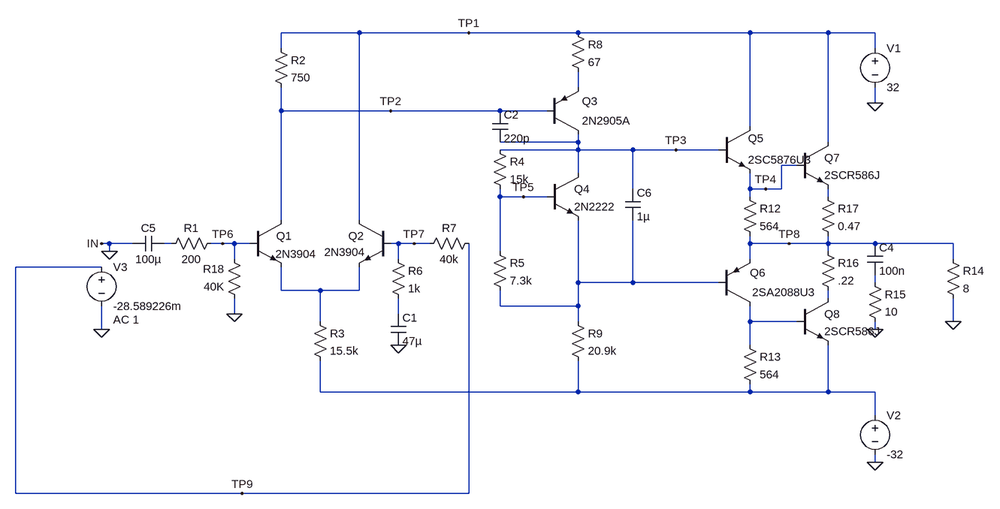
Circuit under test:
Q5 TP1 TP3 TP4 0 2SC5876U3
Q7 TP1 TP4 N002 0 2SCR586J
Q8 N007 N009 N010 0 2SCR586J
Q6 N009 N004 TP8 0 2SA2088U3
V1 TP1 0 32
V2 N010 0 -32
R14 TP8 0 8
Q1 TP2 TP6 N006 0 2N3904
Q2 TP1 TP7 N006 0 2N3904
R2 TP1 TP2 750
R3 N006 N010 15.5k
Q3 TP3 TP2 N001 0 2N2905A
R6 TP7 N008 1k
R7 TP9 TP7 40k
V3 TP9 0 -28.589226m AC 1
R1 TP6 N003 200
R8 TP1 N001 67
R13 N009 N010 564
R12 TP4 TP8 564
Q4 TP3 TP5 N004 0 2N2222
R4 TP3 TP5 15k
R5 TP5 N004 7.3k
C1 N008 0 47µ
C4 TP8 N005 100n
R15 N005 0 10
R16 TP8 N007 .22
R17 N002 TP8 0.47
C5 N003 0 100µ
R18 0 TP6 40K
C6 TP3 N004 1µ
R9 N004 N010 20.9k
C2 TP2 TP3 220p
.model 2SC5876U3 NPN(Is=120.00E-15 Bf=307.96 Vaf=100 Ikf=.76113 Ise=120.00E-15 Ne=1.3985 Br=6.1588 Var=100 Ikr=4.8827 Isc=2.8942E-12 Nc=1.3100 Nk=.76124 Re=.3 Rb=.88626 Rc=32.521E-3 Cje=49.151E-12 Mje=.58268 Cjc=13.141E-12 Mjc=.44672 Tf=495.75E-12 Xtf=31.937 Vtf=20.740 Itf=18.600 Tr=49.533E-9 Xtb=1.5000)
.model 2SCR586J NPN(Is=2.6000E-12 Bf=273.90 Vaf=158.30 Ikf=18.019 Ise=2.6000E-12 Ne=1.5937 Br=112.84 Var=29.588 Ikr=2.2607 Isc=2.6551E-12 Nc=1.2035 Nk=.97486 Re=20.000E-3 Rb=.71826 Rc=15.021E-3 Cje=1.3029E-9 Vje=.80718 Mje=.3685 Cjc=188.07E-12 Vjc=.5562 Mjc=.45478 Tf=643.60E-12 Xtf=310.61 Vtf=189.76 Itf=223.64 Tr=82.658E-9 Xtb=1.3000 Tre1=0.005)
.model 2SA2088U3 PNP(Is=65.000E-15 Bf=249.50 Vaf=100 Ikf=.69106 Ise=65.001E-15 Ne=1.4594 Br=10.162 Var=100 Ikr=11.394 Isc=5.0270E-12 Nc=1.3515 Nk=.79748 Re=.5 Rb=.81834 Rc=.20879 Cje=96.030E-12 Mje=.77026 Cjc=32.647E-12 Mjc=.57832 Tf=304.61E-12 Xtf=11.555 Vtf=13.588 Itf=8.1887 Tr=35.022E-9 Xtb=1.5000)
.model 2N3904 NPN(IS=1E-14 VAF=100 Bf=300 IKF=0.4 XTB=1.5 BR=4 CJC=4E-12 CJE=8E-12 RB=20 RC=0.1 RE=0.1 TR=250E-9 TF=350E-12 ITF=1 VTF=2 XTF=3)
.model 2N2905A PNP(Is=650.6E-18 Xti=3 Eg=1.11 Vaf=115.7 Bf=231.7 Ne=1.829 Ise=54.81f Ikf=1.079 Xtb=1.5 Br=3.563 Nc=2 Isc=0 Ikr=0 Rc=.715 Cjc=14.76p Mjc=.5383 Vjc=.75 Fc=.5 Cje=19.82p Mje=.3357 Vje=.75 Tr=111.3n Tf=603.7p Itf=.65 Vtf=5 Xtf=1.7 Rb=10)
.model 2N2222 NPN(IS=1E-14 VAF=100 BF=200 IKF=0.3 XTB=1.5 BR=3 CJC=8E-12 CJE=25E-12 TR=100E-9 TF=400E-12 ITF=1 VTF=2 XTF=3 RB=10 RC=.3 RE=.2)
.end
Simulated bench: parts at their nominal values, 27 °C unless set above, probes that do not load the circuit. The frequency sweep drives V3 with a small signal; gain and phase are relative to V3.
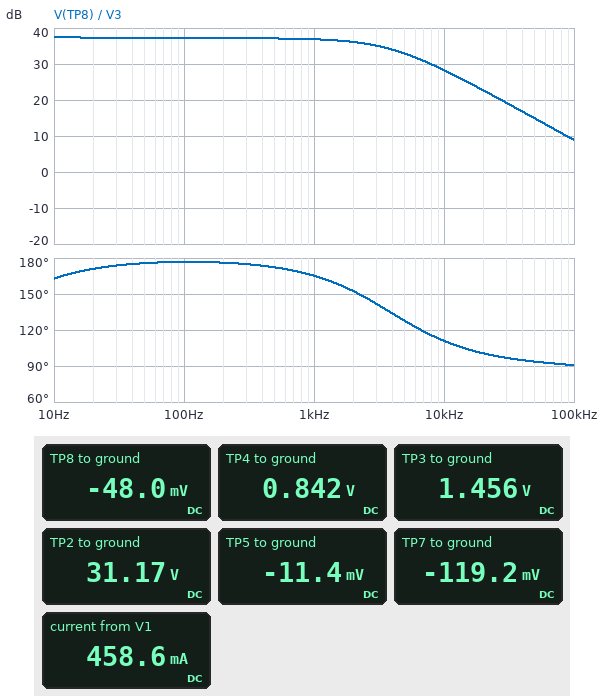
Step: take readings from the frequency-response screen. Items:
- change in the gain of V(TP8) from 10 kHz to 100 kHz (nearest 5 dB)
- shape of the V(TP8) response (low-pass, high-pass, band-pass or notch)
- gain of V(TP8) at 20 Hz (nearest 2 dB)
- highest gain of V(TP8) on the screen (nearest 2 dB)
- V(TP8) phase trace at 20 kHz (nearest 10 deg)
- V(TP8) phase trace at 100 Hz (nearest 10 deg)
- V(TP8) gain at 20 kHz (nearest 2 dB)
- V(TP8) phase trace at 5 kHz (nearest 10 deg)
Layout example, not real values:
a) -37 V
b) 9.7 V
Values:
a) -20 dB
b) low-pass
c) 38 dB
d) 38 dB
e) 100 deg
f) 180 deg
g) 22 dB
h) 130 deg
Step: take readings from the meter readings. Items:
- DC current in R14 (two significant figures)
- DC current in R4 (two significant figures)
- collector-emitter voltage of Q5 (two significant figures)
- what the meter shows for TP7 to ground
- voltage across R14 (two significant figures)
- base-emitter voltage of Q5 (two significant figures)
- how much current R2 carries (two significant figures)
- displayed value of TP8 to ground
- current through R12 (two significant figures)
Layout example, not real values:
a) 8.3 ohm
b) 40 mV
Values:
a) 6.0 mA
b) 98 µA
c) 31 V
d) -119.2 mV
e) 48 mV
f) 610 mV
g) 1.1 mA
h) -48.0 mV
i) 1.6 mA
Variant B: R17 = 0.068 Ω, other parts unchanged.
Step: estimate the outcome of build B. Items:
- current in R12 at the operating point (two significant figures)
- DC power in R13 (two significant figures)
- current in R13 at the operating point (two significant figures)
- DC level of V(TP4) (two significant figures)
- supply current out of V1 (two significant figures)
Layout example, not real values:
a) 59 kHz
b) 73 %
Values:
a) 1.5 mA
b) 960 µW
c) 1.3 mA
d) 850 mV
e) 1.5 A
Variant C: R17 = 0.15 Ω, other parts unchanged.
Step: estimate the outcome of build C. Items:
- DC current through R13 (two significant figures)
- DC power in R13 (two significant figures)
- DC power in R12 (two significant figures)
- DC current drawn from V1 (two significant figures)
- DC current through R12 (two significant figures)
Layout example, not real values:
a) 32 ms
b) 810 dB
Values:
a) 1.3 mA
b) 900 µW
c) 1.3 mW
d) 1.0 A
e) 1.5 mA
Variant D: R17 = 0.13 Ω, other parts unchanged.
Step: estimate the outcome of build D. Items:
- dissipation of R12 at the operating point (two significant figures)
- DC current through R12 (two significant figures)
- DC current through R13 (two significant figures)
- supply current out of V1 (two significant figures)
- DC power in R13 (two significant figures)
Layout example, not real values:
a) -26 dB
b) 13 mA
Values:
a) 1.3 mW
b) 1.5 mA
c) 1.3 mA
d) 1.1 A
e) 910 µW
